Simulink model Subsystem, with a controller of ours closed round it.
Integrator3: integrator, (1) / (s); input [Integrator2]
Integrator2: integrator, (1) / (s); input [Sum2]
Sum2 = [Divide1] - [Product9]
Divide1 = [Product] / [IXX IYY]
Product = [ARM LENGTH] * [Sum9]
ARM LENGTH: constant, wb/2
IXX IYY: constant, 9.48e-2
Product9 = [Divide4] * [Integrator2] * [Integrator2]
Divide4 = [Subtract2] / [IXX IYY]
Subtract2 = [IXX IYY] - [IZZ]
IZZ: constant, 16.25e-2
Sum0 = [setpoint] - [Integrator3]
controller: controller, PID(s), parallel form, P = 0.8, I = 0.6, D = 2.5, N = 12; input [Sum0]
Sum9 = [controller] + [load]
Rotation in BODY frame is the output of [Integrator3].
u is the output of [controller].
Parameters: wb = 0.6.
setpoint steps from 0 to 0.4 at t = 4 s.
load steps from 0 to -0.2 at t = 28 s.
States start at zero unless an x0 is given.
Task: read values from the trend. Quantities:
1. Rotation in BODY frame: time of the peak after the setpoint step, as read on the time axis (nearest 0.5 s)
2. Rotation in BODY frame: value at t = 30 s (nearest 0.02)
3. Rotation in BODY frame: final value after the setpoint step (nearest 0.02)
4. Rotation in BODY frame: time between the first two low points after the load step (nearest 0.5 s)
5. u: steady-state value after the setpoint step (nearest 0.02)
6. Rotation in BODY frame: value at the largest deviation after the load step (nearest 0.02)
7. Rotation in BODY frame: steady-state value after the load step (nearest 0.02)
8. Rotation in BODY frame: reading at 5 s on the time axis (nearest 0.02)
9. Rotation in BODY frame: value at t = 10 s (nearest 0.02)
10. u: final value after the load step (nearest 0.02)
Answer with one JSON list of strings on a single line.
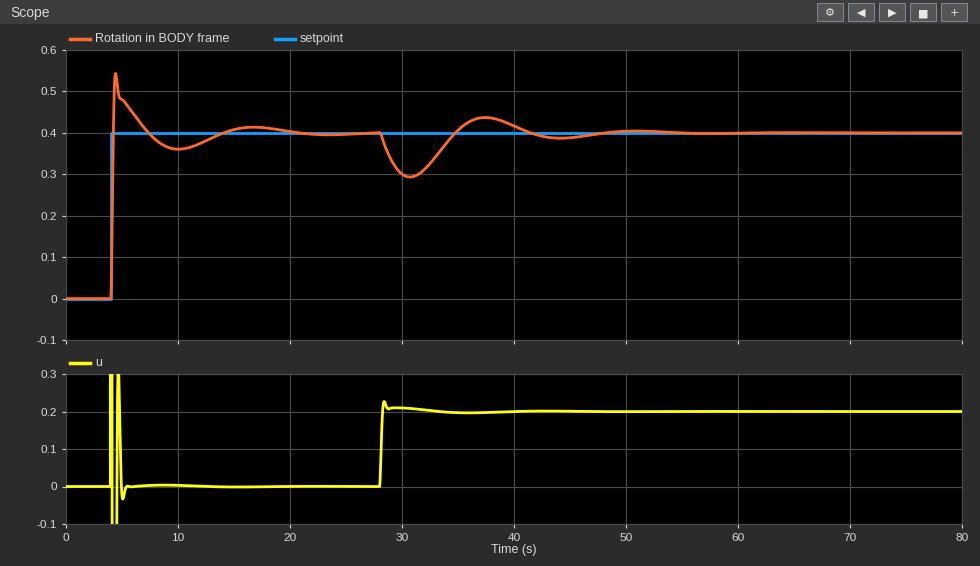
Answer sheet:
["4.5 s", "0.30", "0.40", "13.5 s", "0.00", "0.30", "0.40", "0.48", "0.36", "0.20"]
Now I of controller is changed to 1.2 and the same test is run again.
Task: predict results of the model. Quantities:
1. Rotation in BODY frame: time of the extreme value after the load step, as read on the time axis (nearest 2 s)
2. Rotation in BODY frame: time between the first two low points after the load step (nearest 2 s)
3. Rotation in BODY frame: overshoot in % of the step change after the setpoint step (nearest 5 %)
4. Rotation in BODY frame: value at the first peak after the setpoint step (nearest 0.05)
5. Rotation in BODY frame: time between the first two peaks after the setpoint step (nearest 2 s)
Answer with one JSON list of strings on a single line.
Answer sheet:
["30 s", "10 s", "35 %", "0.55", "8 s"]
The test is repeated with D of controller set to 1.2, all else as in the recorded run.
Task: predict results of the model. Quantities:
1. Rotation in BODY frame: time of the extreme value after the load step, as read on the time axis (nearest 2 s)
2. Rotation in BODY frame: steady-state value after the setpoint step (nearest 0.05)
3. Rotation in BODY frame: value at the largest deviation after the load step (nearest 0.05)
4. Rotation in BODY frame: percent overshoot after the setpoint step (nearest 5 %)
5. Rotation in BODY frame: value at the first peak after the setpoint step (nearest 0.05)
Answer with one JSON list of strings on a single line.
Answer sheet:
["30 s", "0.40", "0.25", "40 %", "0.55"]
